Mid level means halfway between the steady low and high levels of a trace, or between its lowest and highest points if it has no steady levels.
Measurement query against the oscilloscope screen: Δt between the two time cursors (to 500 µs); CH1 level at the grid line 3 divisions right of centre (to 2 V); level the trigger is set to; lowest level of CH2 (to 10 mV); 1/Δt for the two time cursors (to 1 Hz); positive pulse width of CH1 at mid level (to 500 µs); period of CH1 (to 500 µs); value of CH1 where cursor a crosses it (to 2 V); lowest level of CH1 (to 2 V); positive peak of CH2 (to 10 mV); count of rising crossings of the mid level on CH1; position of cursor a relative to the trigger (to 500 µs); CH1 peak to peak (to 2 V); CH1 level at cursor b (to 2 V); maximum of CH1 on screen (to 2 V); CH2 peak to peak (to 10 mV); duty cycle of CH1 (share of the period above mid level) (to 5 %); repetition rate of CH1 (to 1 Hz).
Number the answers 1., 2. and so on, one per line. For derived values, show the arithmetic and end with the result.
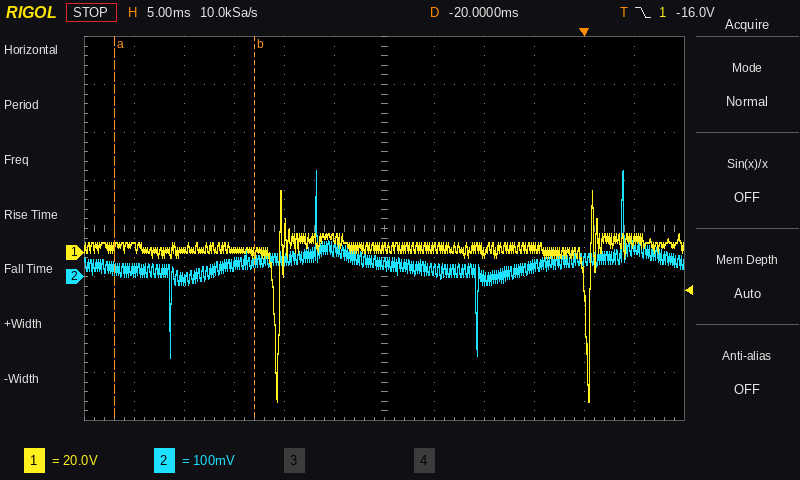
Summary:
1. 14.0 ms
2. 2 V
3. -16.0 V
4. -170 mV
5. 1 / 14.0 ms ≈ 71 Hz
6. 30.5 ms
7. 31.0 ms
8. 2 V
9. -62 V
10. 220 mV
11. 2
12. -47.0 ms
13. 26 V − (-62 V) = 88 V
14. 0 V
15. 26 V
16. 220 mV − (-170 mV) = 390 mV
17. 30.5 ms / 31.0 ms ≈ 98.4 %, so 100 % to the nearest 5 %
18. 1 / 31.0 ms ≈ 32 Hz
